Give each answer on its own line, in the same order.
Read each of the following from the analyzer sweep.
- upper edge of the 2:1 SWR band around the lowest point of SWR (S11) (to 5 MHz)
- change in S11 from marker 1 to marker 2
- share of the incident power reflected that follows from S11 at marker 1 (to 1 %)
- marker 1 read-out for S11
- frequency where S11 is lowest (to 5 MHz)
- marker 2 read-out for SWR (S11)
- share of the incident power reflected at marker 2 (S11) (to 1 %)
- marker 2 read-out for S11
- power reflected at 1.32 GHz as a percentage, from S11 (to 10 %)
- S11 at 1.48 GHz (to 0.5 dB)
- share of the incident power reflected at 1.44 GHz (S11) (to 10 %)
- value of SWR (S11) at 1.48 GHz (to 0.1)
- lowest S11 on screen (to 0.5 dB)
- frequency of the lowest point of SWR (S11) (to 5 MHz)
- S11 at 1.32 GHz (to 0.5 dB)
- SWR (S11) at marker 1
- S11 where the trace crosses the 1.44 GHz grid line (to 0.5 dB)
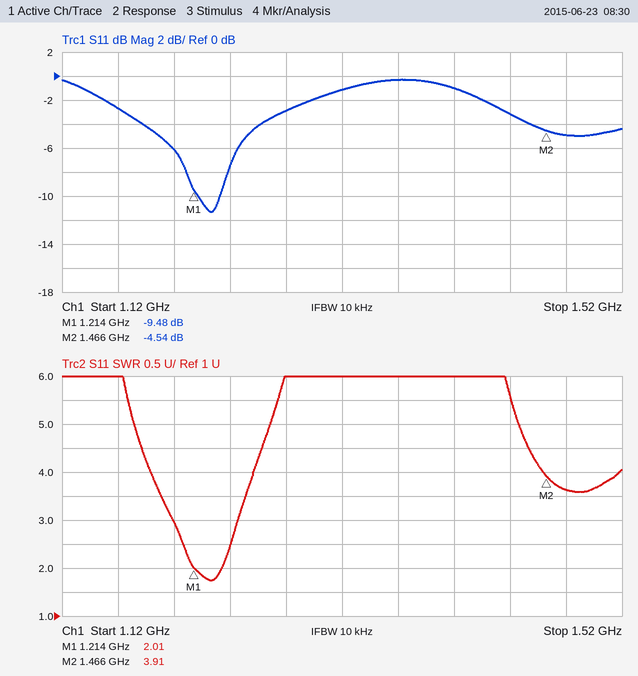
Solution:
1.235 GHz
4.94 dB
11 %
-9.48 dB
1.225 GHz
3.91
35 %
-4.54 dB
80 %
-5.0 dB
50 %
3.6
-11.5 dB
1.225 GHz
-1.0 dB
2.01
-3.0 dB
